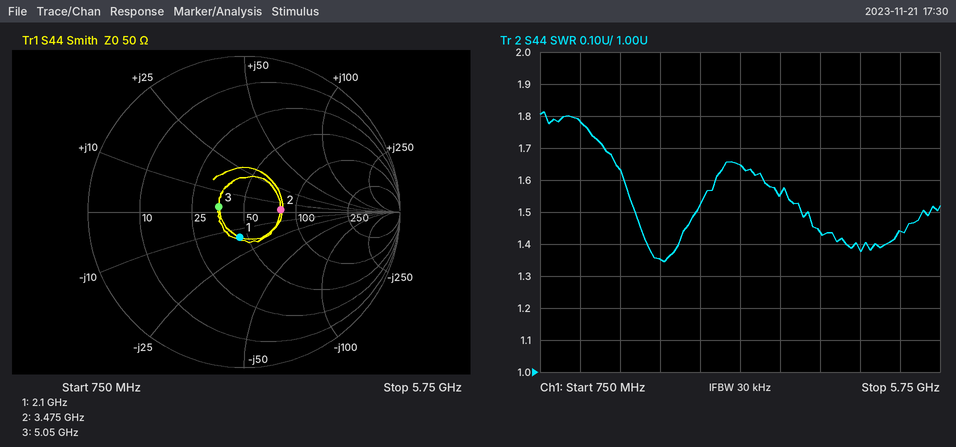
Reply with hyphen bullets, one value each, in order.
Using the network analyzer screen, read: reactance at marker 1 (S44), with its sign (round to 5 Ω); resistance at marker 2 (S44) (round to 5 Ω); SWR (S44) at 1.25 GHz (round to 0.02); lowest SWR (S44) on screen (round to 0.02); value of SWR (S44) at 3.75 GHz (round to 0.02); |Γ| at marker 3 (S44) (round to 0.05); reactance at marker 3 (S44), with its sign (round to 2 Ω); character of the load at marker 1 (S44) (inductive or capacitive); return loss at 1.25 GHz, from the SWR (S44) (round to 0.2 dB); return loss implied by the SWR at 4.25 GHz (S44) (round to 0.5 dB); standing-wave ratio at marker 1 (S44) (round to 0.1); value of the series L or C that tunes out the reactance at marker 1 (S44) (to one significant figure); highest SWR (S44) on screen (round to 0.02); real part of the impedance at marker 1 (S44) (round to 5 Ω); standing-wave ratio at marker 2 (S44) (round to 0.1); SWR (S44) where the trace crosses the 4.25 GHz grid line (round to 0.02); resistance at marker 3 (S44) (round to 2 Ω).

- -15 Ω
- 80 Ω
- 1.78
- 1.34
- 1.56
- 0.15
- +2 Ω
- capacitive
- 11.0 dB
- 15.0 dB
- 1.4
- 1 nH
- 1.82
- 45 Ω
- 1.6
- 1.44
- 36 Ω
